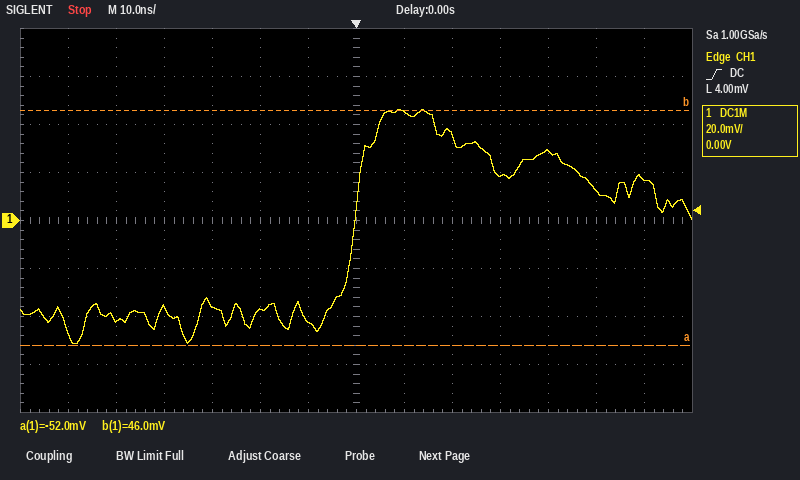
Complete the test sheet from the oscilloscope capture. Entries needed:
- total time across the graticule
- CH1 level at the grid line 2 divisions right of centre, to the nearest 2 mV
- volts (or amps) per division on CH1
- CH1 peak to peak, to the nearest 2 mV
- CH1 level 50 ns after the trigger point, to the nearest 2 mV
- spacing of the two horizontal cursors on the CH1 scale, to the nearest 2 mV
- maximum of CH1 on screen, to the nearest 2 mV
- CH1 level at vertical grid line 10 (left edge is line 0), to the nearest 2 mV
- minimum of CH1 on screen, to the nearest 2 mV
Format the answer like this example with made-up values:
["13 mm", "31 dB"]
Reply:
["140 ns", "36 mV", "20 mV", "98 mV", "12 mV", "98 mV", "46 mV", "18 mV", "-52 mV"]
